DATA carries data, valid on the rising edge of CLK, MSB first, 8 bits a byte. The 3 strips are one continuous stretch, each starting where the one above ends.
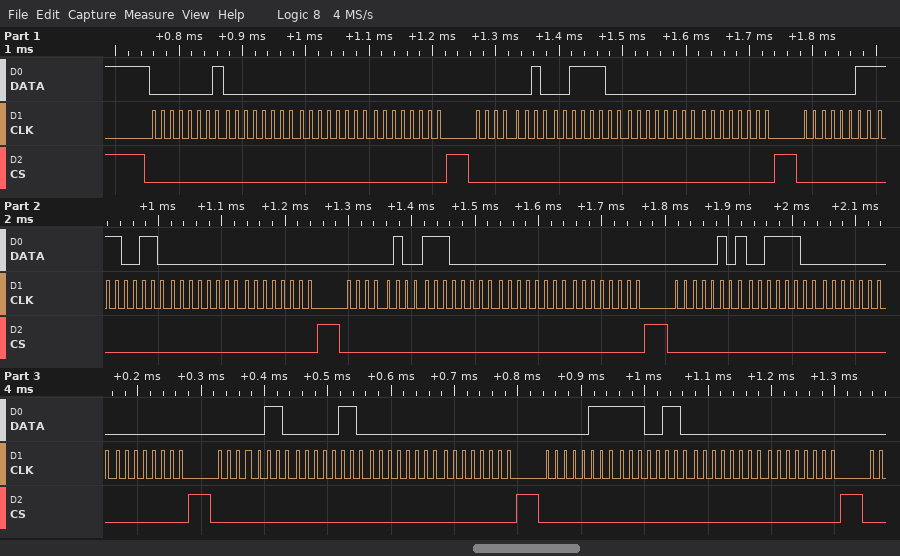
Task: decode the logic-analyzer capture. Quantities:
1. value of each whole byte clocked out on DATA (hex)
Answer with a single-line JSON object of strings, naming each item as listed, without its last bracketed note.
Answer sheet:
{"value of each whole byte clocked out on DATA": "01 00 00 00 02 3C 00 00 03 E6 00 00 04 E0 00 00 05 3C 00 00 06 06 00 00 07 E6 00 00"}
